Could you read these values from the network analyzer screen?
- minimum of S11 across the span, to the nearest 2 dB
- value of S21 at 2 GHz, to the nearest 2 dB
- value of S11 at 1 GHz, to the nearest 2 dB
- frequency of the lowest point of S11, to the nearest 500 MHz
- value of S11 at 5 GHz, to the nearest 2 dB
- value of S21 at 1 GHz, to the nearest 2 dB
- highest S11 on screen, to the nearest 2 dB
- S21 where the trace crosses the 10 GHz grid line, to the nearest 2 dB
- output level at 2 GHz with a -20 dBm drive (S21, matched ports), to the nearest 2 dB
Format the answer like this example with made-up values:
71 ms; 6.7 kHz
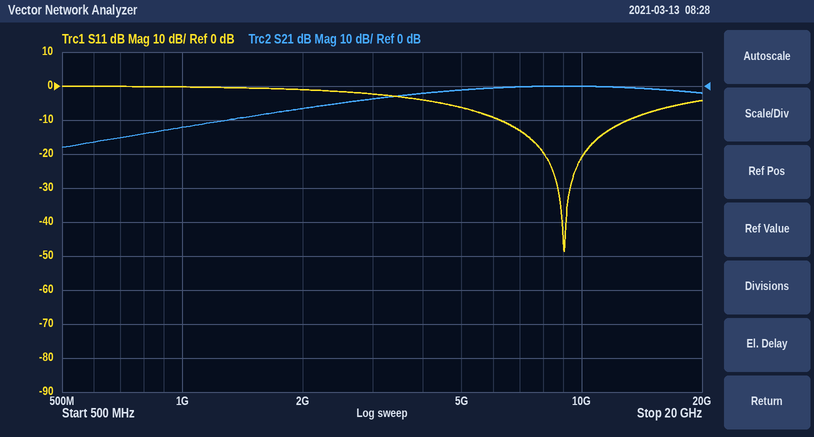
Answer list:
-48 dB; -6 dB; 0 dB; 9.0 GHz; -6 dB; -12 dB; 0 dB; 0 dB; -26 dBm
